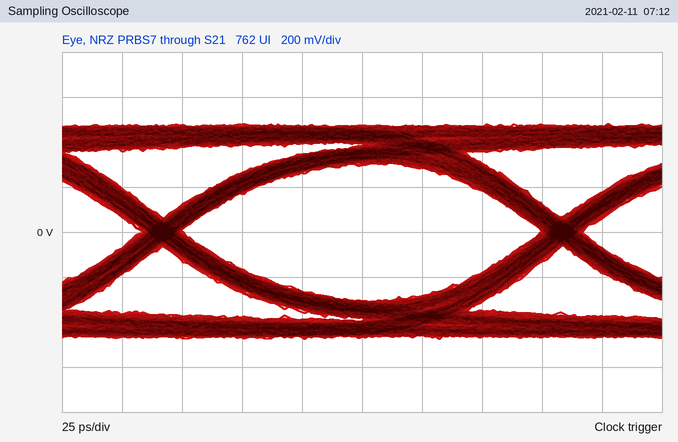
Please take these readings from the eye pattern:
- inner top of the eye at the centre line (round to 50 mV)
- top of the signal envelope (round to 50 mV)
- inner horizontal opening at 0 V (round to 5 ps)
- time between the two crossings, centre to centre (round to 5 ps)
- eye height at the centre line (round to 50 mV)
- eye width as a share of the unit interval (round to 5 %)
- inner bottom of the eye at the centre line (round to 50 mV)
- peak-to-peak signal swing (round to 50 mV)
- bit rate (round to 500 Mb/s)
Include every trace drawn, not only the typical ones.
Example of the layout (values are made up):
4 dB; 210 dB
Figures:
300 mV; 500 mV; 150 ps; 165 ps; 600 mV; 90 %; -300 mV; 950 mV; 6.0 Gb/s
